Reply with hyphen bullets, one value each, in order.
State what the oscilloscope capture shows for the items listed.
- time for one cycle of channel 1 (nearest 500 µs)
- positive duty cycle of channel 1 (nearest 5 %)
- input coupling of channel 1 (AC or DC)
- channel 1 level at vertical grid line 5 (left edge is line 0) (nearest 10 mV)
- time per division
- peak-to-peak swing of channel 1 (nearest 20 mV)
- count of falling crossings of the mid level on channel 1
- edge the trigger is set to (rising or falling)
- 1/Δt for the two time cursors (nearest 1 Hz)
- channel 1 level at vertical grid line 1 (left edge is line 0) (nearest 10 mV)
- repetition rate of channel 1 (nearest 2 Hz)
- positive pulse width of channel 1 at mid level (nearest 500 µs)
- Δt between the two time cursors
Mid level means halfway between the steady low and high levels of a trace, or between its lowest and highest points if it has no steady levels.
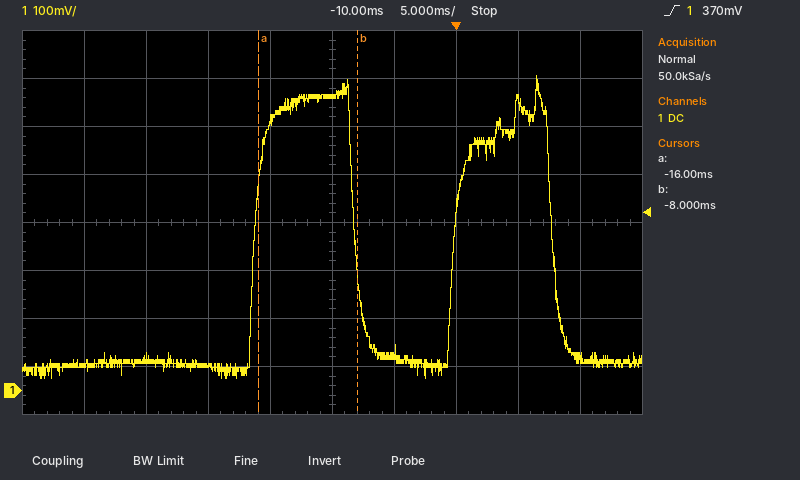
- 16.0 ms
- 50 %
- DC
- 610 mV
- 5 ms
- 640 mV
- 2
- rising
- 125 Hz
- 60 mV
- 62 Hz
- 8.0 ms
- 8.0 ms
